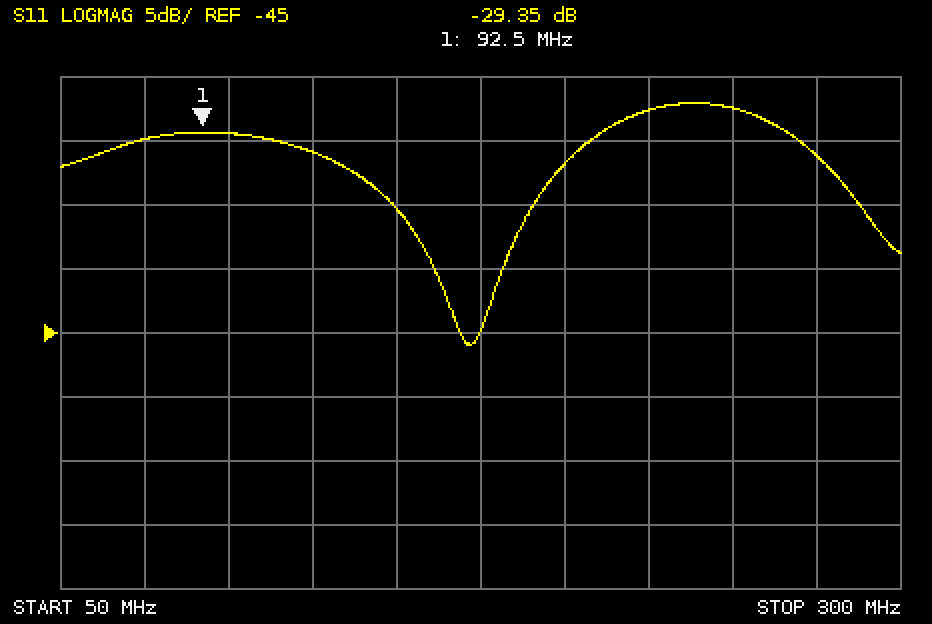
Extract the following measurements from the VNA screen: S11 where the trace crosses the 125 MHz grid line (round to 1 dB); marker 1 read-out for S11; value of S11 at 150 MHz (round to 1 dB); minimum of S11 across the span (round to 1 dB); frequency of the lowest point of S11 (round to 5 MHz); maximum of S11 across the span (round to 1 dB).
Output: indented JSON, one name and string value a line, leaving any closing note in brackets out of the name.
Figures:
{
  "S11 where the trace crosses the 125 MHz grid line": "-31 dB",
  "marker 1 read-out for S11": "-29.35 dB",
  "value of S11 at 150 MHz": "-35 dB",
  "minimum of S11 across the span": "-46 dB",
  "frequency of the lowest point of S11": "170 MHz",
  "maximum of S11 across the span": "-27 dB"
}
